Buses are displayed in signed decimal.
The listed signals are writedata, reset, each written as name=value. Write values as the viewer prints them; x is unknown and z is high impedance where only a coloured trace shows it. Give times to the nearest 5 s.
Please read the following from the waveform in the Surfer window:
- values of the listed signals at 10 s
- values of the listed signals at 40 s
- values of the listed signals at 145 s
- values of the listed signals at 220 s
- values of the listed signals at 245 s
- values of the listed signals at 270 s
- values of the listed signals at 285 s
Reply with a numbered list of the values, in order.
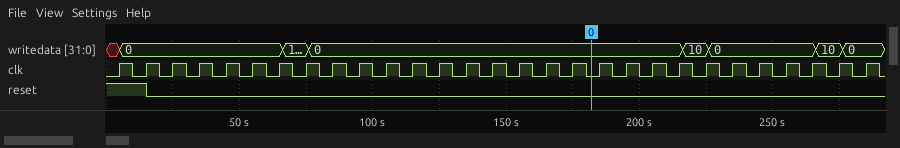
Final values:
1. writedata=0, reset=1
2. writedata=0, reset=0
3. writedata=0, reset=0
4. writedata=10, reset=0
5. writedata=0, reset=0
6. writedata=10, reset=0
7. writedata=0, reset=0
